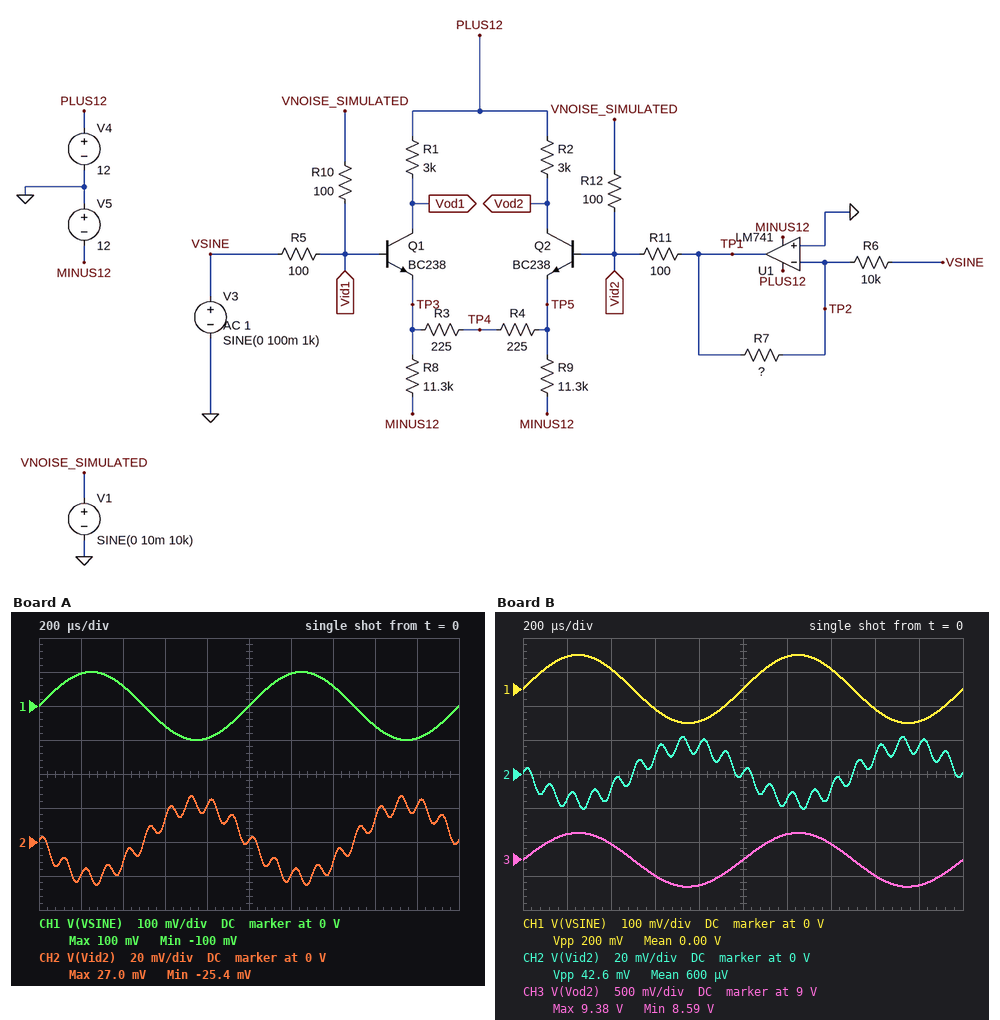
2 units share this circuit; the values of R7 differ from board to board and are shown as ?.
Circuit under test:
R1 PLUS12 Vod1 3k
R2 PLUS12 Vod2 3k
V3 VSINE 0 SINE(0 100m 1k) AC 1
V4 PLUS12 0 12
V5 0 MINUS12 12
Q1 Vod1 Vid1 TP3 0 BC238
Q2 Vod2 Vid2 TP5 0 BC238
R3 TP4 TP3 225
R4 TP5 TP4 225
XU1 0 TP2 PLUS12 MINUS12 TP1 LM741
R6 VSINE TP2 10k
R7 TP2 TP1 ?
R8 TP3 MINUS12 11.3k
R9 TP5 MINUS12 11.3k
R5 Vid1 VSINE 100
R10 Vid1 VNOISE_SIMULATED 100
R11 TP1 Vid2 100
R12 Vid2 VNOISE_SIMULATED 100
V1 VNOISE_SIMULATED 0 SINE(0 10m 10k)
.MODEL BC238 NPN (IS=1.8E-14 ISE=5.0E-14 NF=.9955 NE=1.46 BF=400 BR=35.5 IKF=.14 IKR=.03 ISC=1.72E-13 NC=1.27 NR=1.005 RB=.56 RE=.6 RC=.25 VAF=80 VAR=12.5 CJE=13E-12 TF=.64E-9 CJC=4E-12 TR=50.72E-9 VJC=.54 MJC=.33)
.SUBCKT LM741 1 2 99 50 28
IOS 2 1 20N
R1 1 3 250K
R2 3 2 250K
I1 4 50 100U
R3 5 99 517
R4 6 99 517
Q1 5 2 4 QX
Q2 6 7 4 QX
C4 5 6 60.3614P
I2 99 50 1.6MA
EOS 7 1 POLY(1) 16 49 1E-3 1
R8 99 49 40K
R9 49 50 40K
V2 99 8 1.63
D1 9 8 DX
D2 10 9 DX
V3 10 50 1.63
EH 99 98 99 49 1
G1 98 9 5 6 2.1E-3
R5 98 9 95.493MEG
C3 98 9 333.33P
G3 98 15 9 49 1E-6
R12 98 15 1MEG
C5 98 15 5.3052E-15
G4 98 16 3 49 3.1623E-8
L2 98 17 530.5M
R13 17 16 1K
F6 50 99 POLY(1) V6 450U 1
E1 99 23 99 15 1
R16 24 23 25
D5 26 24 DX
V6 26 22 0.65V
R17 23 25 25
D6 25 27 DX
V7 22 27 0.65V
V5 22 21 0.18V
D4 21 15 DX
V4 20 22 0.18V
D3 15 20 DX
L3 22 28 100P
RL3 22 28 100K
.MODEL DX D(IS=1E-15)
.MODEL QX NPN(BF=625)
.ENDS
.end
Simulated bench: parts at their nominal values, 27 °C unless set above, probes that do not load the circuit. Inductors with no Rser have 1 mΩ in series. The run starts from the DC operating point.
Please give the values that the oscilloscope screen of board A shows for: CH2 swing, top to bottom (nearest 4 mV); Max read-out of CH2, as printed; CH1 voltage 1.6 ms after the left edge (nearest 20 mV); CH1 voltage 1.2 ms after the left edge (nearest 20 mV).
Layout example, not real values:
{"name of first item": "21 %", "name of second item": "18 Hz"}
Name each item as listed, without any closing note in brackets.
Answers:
{"CH2 swing, top to bottom": "52 mV", "Max read-out of CH2, as printed": "27.0 mV", "CH1 voltage 1.6 ms after the left edge": "-60 mV", "CH1 voltage 1.2 ms after the left edge": "100 mV"}
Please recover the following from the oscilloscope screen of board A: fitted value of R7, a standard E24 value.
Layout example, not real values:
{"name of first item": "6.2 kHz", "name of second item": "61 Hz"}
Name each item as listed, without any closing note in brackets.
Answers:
{"fitted value of R7, a standard E24 value": "4.3 kΩ"}
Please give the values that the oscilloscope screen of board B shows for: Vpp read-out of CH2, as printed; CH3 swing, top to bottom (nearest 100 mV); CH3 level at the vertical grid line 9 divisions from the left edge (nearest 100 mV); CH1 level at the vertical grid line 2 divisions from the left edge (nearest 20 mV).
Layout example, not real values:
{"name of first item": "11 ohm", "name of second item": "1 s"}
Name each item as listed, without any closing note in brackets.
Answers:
{"Vpp read-out of CH2, as printed": "42.6 mV", "CH3 swing, top to bottom": "800 mV", "CH3 level at the vertical grid line 9 divisions from the left edge": "8.6 V", "CH1 level at the vertical grid line 2 divisions from the left edge": "60 mV"}
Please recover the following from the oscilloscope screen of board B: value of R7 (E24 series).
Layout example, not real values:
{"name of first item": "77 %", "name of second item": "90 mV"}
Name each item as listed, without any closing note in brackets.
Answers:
{"value of R7": "3.3 kΩ"}
